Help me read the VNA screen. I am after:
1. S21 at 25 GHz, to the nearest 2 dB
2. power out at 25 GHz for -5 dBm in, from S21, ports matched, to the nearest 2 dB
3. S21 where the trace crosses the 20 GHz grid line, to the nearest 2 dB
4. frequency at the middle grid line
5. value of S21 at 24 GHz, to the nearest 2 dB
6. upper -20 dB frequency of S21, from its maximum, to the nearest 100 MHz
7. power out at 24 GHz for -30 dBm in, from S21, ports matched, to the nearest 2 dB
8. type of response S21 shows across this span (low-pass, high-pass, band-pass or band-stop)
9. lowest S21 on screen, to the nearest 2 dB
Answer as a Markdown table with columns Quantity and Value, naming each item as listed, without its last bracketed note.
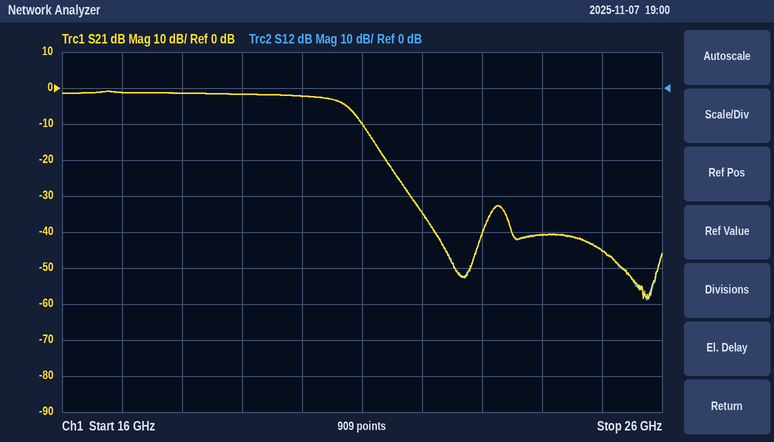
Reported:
| Quantity | Value |
|---|---|
| S21 at 25 GHz, to the nearest 2 dB | -46 dB |
| power out at 25 GHz for -5 dBm in, from S21, ports matched, to the nearest 2 dB | -50 dBm |
| S21 where the trace crosses the 20 GHz grid line, to the nearest 2 dB | -2 dB |
| frequency at the middle grid line | 21 GHz |
| value of S21 at 24 GHz, to the nearest 2 dB | -40 dB |
| upper -20 dB frequency of S21, from its maximum, to the nearest 100 MHz | 21.4 GHz |
| power out at 24 GHz for -30 dBm in, from S21, ports matched, to the nearest 2 dB | -70 dBm |
| type of response S21 shows across this span | low-pass |
| lowest S21 on screen, to the nearest 2 dB | -58 dB |
